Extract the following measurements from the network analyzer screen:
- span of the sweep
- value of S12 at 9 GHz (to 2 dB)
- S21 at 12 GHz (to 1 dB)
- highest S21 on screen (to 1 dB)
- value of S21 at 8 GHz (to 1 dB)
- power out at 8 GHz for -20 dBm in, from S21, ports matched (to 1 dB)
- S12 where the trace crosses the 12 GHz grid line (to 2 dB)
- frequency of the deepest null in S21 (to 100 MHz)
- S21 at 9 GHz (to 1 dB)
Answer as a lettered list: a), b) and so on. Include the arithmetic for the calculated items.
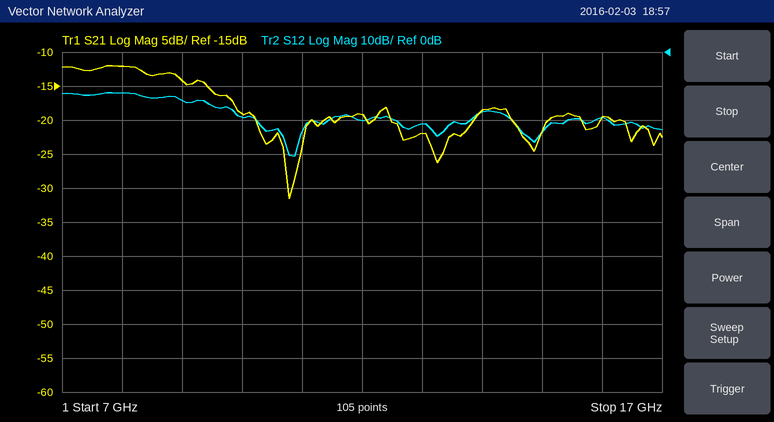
a) 10 GHz
b) -14 dB
c) -19 dB
d) -12 dB
e) -12 dB
f) -20 dBm + (-12 dB) = -32 dBm
g) -20 dB
h) 10.8 GHz
i) -14 dB
